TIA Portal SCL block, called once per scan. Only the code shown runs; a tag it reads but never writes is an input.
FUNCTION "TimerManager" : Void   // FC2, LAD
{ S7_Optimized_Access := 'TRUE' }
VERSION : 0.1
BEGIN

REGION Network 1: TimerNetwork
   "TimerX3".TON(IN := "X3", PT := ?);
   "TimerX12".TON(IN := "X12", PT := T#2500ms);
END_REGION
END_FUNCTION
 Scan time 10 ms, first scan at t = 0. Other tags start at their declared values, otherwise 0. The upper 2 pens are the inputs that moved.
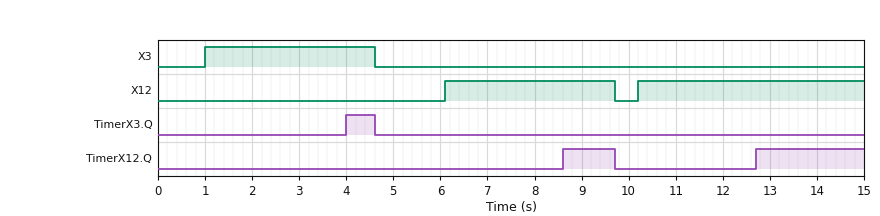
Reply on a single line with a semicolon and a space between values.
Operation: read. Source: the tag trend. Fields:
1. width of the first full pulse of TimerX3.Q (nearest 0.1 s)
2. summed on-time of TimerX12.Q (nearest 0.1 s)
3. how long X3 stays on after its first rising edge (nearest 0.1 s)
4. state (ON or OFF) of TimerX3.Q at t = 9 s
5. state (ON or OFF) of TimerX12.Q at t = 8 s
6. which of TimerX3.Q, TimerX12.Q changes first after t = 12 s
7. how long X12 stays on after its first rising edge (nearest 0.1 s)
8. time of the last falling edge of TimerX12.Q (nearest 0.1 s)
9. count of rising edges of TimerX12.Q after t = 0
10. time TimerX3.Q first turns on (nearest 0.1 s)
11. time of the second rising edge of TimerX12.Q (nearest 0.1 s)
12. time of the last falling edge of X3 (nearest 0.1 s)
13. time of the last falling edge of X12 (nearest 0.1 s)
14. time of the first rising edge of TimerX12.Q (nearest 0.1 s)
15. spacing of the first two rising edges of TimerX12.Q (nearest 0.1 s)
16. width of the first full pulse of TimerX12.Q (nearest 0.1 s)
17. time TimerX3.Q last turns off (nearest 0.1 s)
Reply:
0.6 s; 3.4 s; 3.6 s; OFF; OFF; TimerX12.Q; 3.6 s; 9.7 s; 2; 4.0 s; 12.7 s; 4.6 s; 9.7 s; 8.6 s; 4.1 s; 1.1 s; 4.6 s
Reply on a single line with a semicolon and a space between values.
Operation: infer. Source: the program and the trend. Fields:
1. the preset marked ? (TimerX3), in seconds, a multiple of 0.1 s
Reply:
3.0 s
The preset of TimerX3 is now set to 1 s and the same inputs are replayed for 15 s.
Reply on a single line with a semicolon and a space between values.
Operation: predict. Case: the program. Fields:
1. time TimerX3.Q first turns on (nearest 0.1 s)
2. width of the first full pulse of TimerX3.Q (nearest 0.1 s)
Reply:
2.0 s; 2.6 s
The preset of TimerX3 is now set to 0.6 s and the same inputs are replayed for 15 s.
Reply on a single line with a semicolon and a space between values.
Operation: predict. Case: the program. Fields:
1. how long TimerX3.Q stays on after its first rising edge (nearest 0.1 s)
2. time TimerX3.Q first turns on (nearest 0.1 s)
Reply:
3.0 s; 1.6 s
